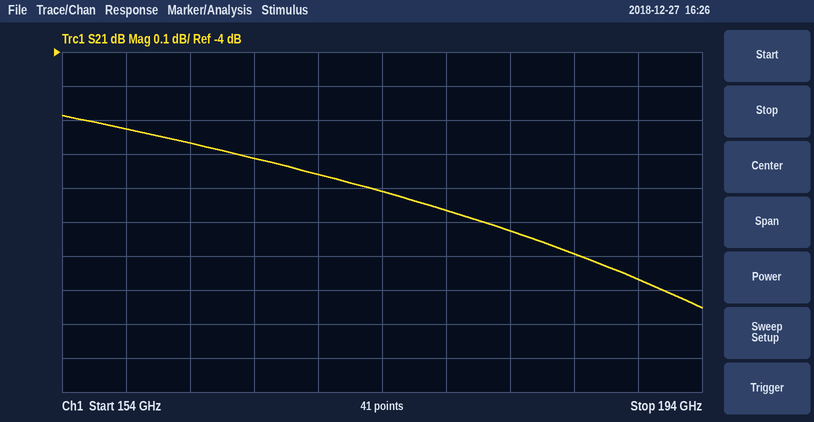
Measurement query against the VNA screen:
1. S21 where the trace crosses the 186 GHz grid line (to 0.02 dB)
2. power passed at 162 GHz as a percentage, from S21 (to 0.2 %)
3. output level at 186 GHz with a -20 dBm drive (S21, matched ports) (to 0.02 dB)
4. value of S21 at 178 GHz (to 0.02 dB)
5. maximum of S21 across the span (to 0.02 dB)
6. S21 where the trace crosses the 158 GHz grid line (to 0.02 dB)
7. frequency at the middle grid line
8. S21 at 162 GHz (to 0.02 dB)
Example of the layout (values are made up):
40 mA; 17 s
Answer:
-4.60 dB; 37.4 %; -24.60 dBm; -4.46 dB; -4.18 dB; -4.22 dB; 174 GHz; -4.26 dB
